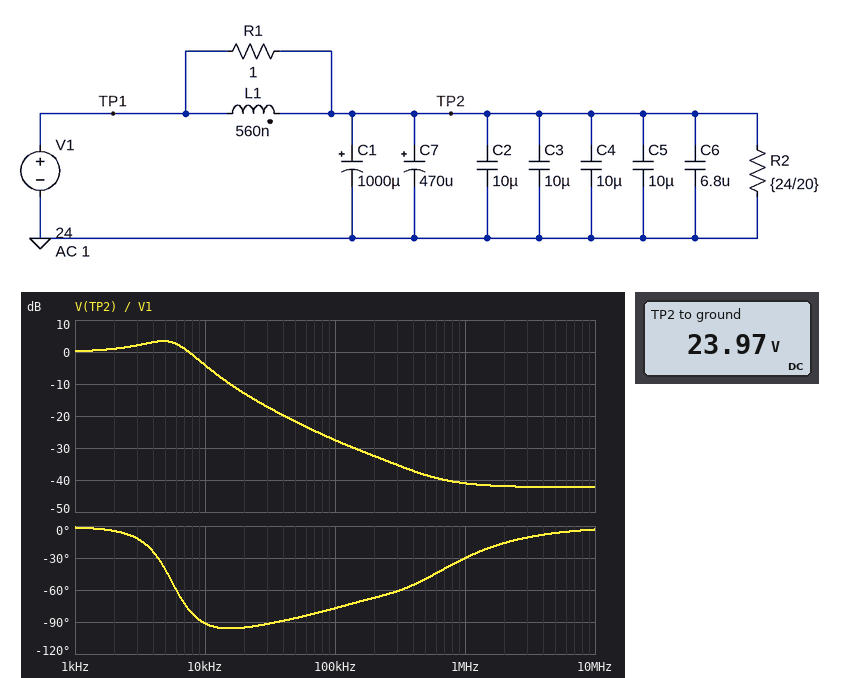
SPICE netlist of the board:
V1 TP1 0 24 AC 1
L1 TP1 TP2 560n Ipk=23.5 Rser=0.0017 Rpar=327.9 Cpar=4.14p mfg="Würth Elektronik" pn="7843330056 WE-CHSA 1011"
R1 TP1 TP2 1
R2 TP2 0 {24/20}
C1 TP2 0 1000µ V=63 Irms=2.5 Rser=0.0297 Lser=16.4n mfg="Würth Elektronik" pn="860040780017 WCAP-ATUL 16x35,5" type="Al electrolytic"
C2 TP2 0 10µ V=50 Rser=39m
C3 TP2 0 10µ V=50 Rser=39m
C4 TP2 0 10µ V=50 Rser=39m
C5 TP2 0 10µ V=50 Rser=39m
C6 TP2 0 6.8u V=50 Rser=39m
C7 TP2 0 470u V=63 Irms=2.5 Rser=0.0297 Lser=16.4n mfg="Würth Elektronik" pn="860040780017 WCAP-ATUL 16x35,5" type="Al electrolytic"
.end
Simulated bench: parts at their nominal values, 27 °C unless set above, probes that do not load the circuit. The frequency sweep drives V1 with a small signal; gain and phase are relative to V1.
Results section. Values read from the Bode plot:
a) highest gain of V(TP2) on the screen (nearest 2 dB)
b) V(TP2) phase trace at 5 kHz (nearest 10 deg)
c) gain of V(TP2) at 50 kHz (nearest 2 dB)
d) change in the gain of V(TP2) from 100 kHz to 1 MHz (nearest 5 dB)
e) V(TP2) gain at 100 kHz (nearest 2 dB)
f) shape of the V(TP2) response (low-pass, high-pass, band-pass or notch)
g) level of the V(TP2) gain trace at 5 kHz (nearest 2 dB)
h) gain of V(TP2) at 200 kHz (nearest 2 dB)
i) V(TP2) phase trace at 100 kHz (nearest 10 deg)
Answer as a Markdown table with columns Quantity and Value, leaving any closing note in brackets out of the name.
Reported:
| Quantity | Value |
|---|---|
| highest gain of V(TP2) on the screen | 4 dB |
| V(TP2) phase trace at 5 kHz | -40 deg |
| gain of V(TP2) at 50 kHz | -22 dB |
| change in the gain of V(TP2) from 100 kHz to 1 MHz | -15 dB |
| V(TP2) gain at 100 kHz | -28 dB |
| shape of the V(TP2) response | low-pass |
| level of the V(TP2) gain trace at 5 kHz | 4 dB |
| gain of V(TP2) at 200 kHz | -32 dB |
| V(TP2) phase trace at 100 kHz | -80 deg |
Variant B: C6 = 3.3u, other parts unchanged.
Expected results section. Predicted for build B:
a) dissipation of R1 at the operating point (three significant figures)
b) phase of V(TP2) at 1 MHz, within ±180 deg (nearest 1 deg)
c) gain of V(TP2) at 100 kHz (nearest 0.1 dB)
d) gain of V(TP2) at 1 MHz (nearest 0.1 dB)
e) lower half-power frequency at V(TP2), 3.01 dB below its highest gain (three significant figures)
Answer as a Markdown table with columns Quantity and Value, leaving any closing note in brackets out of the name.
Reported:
| Quantity | Value |
|---|---|
| dissipation of R1 at the operating point | 1.15 mW |
| phase of V(TP2) at 1 MHz, within ±180 deg | -32 deg |
| gain of V(TP2) at 100 kHz | -27.4 dB |
| gain of V(TP2) at 1 MHz | -40.4 dB |
| lower half-power frequency at V(TP2), 3.01 dB below its highest gain | 1.21 kHz |
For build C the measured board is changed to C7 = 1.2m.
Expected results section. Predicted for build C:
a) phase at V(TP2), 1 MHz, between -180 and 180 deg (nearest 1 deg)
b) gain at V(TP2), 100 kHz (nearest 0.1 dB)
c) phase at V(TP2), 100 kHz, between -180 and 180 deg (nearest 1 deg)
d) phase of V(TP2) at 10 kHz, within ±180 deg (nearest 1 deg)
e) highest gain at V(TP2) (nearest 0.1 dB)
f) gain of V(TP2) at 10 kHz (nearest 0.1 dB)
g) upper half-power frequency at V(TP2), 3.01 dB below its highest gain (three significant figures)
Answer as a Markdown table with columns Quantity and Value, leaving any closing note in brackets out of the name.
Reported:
| Quantity | Value |
|---|---|
| phase at V(TP2), 1 MHz, between -180 and 180 deg | -30 deg |
| gain at V(TP2), 100 kHz | -27.4 dB |
| phase at V(TP2), 100 kHz, between -180 and 180 deg | -76 deg |
| phase of V(TP2) at 10 kHz, within ±180 deg | -85 deg |
| highest gain at V(TP2) | 2.7 dB |
| gain of V(TP2) at 10 kHz | -6.3 dB |
| upper half-power frequency at V(TP2), 3.01 dB below its highest gain | 6.03 kHz |
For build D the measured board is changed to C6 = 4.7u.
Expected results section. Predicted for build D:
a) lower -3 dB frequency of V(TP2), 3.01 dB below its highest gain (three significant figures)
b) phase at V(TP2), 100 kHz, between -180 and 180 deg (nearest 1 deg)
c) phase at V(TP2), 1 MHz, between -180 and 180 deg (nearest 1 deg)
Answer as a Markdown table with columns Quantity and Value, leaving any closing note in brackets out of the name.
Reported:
| Quantity | Value |
|---|---|
| lower -3 dB frequency of V(TP2), 3.01 dB below its highest gain | 1.22 kHz |
| phase at V(TP2), 100 kHz, between -180 and 180 deg | -76 deg |
| phase at V(TP2), 1 MHz, between -180 and 180 deg | -31 deg |
